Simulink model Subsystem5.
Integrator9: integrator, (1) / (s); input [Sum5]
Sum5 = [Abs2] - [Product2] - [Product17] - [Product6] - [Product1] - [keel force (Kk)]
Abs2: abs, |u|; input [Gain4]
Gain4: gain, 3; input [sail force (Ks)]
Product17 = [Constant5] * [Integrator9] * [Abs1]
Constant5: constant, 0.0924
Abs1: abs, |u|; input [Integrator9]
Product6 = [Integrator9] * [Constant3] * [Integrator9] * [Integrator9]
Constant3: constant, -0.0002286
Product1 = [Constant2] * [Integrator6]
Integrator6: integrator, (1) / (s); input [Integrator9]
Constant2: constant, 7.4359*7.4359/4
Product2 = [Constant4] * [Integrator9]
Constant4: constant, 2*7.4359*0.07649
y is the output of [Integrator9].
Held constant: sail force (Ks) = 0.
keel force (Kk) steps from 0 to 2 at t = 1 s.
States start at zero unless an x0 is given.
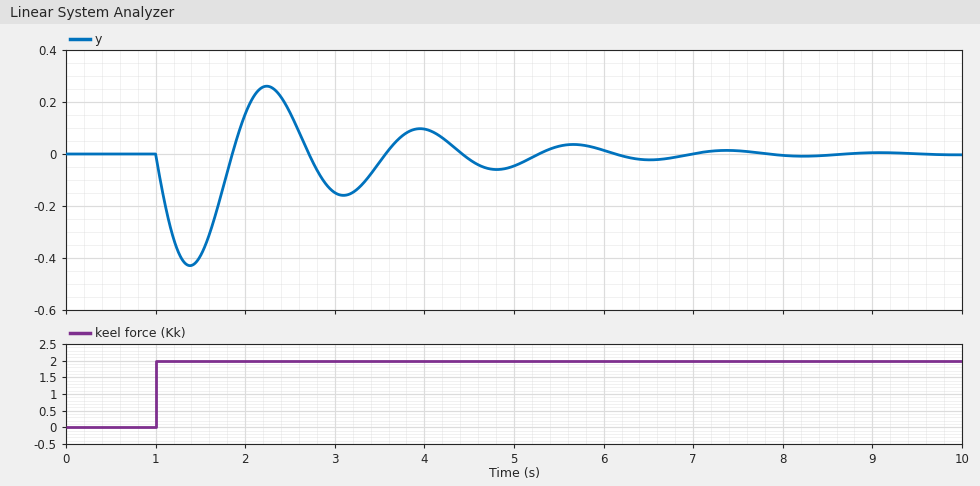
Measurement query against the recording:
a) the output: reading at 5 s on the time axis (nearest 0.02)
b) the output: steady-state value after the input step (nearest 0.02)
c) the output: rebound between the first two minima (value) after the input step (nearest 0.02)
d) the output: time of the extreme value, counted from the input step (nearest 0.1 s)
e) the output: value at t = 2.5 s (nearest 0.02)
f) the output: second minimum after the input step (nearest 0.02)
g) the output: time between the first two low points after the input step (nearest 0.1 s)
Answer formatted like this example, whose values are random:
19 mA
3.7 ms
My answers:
-0.04
0.00
0.26
0.4 s
0.16
-0.16
1.7 s
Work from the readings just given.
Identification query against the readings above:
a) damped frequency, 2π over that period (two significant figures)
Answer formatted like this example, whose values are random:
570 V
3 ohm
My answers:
3.7 rad/s
